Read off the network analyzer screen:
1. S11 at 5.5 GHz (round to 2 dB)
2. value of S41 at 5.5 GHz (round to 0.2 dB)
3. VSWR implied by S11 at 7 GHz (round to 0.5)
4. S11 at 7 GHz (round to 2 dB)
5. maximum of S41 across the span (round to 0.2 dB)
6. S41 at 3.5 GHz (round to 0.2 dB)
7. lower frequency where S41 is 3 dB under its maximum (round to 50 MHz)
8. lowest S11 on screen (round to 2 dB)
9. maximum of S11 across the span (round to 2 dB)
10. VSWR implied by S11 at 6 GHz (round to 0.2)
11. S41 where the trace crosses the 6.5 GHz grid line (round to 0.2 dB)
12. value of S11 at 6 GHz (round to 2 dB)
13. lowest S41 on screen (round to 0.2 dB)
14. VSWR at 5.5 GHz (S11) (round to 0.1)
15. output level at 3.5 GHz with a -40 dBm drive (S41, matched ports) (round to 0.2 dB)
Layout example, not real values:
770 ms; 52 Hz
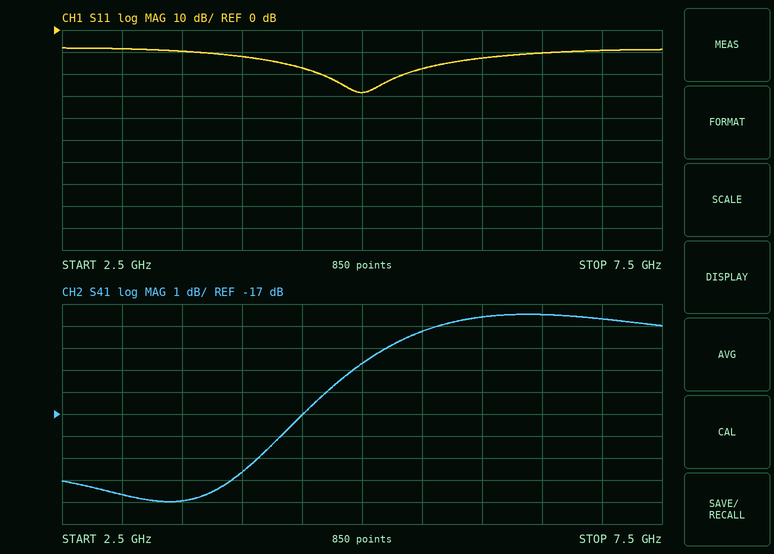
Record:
-18 dB; -13.2 dB; 2.0; -10 dB; -12.4 dB; -21.0 dB; 4.80 GHz; -28 dB; -8 dB; 1.6; -12.4 dB; -12 dB; -21.0 dB; 1.3; -61.0 dBm
